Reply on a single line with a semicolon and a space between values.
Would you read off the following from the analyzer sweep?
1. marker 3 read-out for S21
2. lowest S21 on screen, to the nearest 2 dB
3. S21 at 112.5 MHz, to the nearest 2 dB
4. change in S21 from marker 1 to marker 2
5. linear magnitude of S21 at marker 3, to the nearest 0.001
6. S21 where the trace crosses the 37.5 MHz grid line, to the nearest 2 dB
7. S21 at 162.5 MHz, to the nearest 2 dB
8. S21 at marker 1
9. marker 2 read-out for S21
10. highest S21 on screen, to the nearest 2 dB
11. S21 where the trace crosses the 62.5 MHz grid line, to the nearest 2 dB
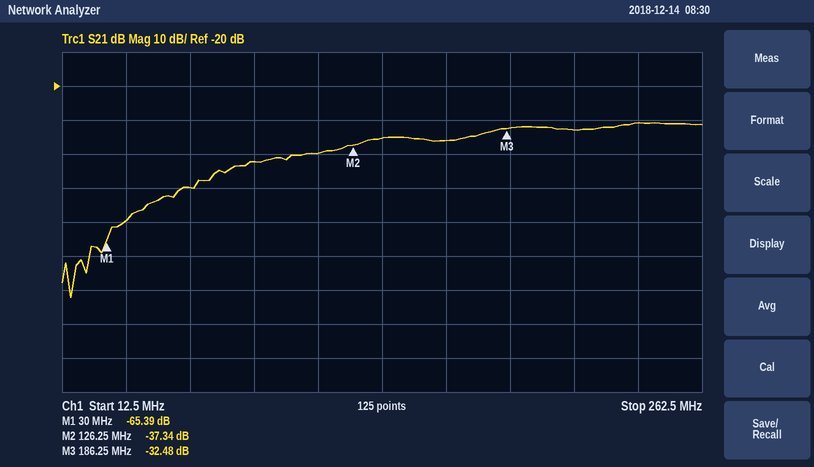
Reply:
-32.48 dB; -82 dB; -40 dB; 28.05 dB; 0.024; -60 dB; -36 dB; -65.39 dB; -37.34 dB; -30 dB; -50 dB
